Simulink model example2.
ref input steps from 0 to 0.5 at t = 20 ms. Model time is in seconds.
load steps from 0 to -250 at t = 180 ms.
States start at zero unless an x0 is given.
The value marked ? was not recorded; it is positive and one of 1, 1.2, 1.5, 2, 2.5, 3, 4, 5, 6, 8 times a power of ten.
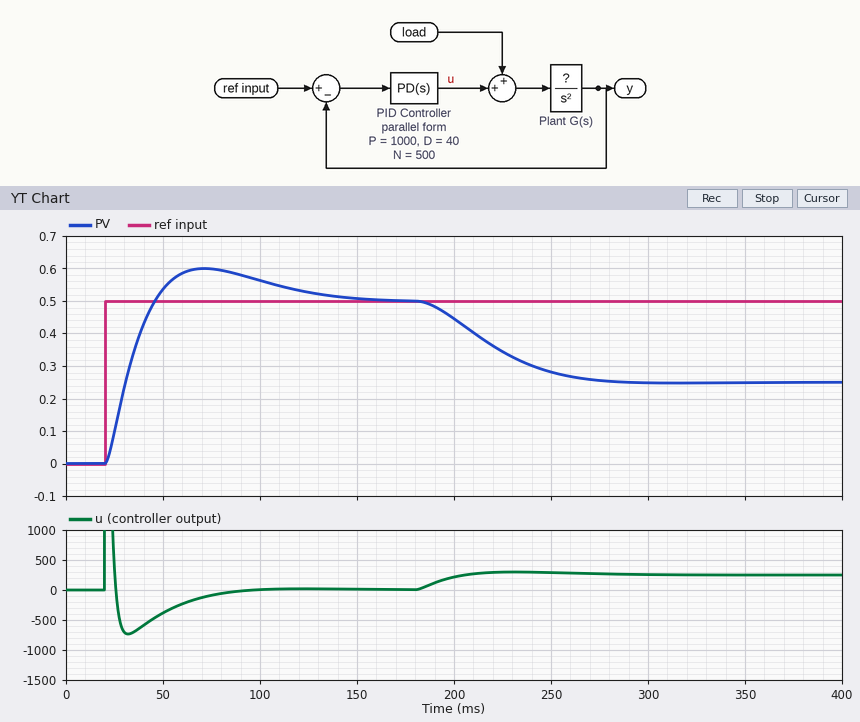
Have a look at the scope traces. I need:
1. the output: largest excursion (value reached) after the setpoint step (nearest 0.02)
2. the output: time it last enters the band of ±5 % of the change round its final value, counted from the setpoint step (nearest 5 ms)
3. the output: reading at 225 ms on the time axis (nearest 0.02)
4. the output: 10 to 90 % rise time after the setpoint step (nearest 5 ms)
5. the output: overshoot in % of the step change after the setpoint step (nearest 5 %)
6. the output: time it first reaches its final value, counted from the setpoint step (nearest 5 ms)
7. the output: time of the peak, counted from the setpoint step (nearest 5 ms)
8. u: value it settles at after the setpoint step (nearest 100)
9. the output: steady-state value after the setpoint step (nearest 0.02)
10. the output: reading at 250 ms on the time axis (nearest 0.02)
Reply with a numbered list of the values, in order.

1. 0.60
2. 105 ms
3. 0.34
4. 20 ms
5. 20 %
6. 25 ms
7. 50 ms
8. 0
9. 0.50
10. 0.28
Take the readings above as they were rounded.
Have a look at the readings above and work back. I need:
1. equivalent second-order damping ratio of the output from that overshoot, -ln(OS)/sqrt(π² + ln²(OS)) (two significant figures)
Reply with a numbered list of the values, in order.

1. 0.46
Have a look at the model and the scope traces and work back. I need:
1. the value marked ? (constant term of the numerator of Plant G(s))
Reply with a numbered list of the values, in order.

1. 1.5
